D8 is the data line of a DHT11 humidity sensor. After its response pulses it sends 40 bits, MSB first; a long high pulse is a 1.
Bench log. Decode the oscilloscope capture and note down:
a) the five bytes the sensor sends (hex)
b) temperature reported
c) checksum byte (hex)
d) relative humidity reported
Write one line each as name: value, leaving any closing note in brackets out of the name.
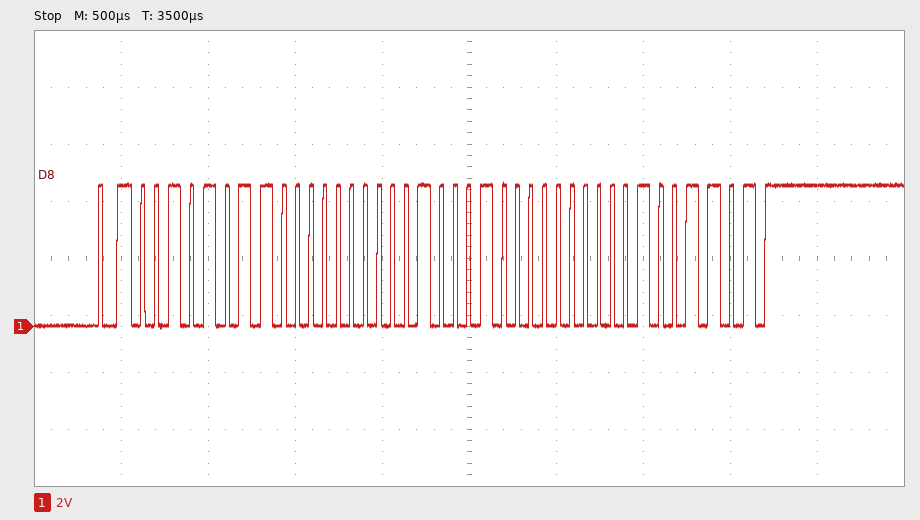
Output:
the five bytes the sensor sends: 2B 00 22 00 4D
temperature reported: 34.0 °C
checksum byte: 0x4D
relative humidity reported: 43 %
